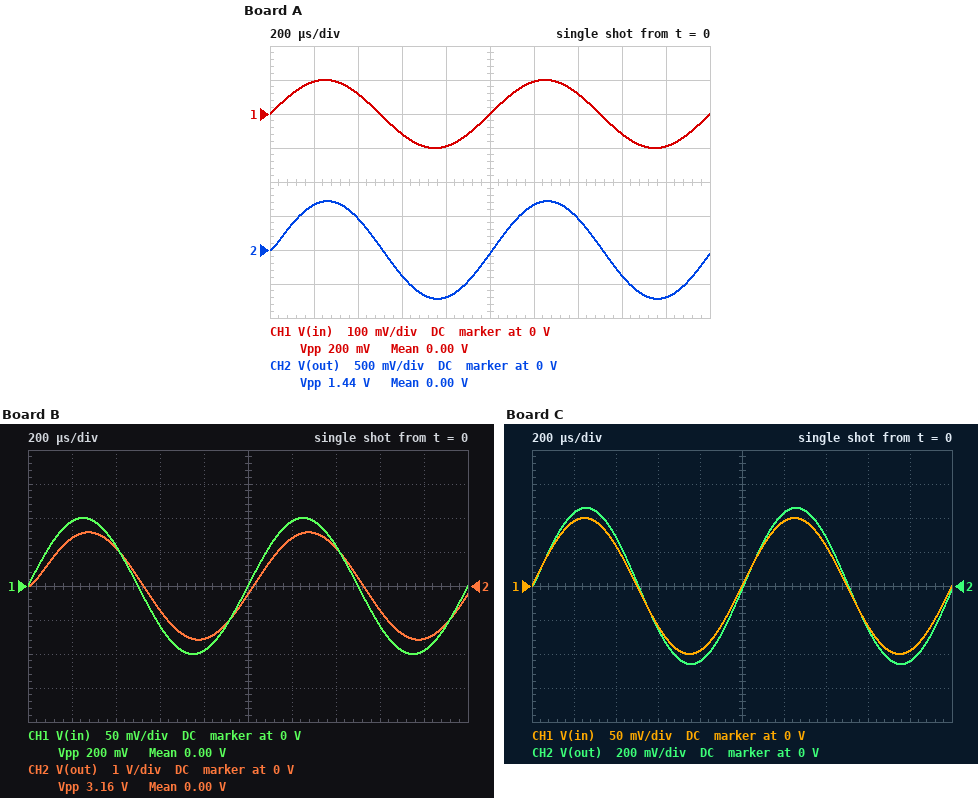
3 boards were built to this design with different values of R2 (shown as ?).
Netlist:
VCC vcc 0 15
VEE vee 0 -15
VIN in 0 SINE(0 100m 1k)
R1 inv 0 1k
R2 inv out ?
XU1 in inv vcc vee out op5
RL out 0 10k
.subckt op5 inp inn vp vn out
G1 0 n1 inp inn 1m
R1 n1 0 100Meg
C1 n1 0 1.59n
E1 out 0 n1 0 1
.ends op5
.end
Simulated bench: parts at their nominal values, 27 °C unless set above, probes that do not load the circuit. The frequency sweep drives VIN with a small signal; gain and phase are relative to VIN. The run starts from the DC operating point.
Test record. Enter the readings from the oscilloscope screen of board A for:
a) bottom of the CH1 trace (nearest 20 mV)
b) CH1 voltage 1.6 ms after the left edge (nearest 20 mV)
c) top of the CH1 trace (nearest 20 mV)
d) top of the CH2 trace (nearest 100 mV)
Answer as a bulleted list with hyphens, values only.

- -100 mV
- -60 mV
- 100 mV
- 700 mV
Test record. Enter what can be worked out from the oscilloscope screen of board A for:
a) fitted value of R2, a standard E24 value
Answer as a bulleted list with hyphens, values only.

- 6.2 kΩ
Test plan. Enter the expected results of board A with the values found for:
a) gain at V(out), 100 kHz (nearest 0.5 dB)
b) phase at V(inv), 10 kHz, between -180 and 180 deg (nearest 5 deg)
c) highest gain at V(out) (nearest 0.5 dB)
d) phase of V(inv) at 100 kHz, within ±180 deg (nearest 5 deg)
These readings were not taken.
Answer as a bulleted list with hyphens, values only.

- 0 dB
- -35 deg
- 17.0 dB
- -80 deg
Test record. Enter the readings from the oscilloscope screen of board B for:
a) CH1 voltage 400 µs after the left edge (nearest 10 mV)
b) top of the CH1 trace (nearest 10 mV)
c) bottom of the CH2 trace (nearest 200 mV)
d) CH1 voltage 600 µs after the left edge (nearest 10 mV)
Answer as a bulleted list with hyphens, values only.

- 60 mV
- 100 mV
- -1.6 V
- -60 mV
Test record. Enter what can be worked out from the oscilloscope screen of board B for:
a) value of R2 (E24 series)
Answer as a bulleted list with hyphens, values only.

- 15 kΩ
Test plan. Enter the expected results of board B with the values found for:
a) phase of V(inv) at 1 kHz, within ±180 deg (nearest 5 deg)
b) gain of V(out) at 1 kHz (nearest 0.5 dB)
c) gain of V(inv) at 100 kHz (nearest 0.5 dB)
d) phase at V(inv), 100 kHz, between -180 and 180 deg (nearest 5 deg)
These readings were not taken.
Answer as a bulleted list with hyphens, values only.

- -10 deg
- 24.0 dB
- -24.0 dB
- -85 deg
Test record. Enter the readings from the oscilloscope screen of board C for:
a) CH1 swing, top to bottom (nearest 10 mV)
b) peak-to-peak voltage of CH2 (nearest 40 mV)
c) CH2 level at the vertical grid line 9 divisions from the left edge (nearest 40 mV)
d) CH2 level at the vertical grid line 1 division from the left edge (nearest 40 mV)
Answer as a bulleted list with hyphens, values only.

- 200 mV
- 920 mV
- -440 mV
- 440 mV
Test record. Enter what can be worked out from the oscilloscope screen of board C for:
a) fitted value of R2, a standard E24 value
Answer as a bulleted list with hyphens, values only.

- 3.6 kΩ
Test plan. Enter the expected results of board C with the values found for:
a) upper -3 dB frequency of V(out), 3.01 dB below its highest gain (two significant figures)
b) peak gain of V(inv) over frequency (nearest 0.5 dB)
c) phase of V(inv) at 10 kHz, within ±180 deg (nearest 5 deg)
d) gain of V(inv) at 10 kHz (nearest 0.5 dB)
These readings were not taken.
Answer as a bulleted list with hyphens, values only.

- 22 kHz
- 0 dB
- -25 deg
- -1.0 dB
